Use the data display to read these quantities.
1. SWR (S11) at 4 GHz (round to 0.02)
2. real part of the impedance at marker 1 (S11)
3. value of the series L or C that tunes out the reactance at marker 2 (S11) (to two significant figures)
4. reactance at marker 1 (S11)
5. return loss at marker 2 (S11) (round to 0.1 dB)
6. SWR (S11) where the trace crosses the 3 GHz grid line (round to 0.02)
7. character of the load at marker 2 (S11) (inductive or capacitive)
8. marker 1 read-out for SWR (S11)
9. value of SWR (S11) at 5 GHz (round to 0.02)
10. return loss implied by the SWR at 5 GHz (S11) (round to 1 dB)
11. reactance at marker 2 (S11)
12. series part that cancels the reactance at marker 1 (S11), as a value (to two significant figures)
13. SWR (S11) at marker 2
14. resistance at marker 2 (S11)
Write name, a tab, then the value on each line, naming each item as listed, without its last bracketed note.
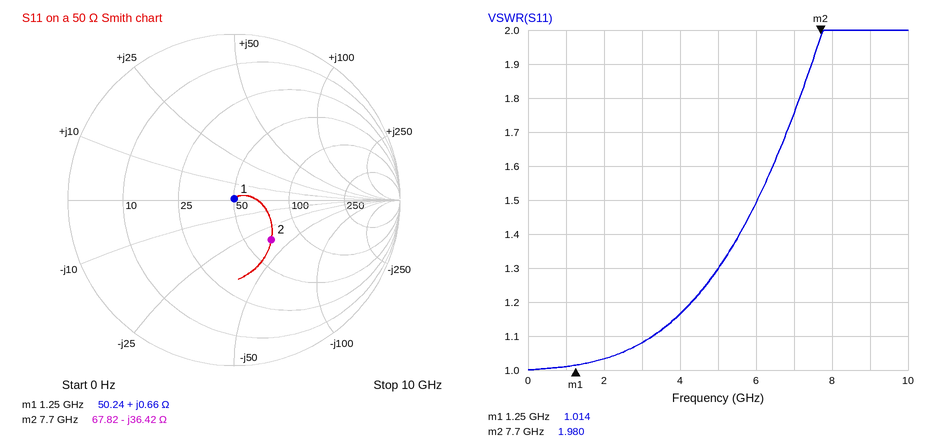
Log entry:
SWR (S11) at 4 GHz	1.16
real part of the impedance at marker 1	50.24 Ω
value of the series L or C that tunes out the reactance at marker 2 (S11)	750 pH
reactance at marker 1	+0.66 Ω
return loss at marker 2 (S11)	9.7 dB
SWR (S11) where the trace crosses the 3 GHz grid line	1.08
character of the load at marker 2 (S11)	capacitive
marker 1 read-out for SWR	1.014
value of SWR (S11) at 5 GHz	1.30
return loss implied by the SWR at 5 GHz (S11)	18 dB
reactance at marker 2	-36.42 Ω
series part that cancels the reactance at marker 1 (S11), as a value	190 pF
SWR (S11) at marker 2	1.980
resistance at marker 2	67.82 Ω
